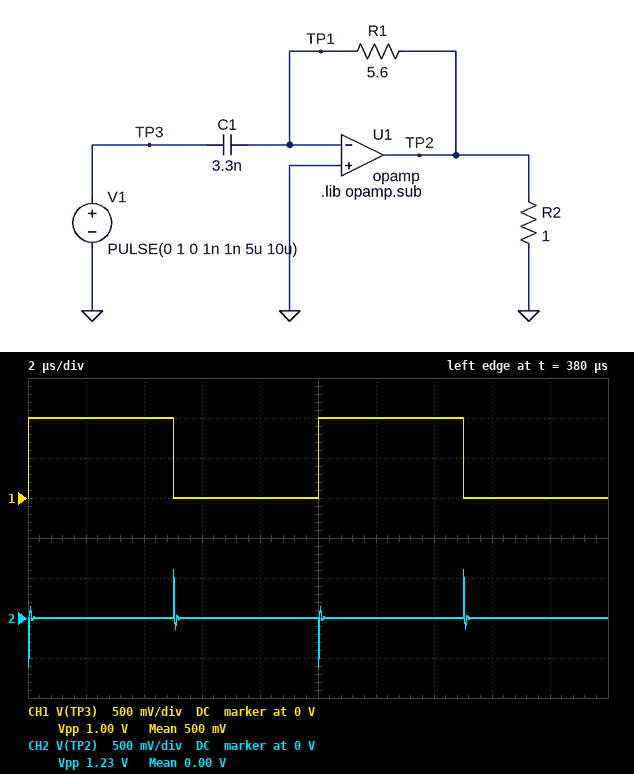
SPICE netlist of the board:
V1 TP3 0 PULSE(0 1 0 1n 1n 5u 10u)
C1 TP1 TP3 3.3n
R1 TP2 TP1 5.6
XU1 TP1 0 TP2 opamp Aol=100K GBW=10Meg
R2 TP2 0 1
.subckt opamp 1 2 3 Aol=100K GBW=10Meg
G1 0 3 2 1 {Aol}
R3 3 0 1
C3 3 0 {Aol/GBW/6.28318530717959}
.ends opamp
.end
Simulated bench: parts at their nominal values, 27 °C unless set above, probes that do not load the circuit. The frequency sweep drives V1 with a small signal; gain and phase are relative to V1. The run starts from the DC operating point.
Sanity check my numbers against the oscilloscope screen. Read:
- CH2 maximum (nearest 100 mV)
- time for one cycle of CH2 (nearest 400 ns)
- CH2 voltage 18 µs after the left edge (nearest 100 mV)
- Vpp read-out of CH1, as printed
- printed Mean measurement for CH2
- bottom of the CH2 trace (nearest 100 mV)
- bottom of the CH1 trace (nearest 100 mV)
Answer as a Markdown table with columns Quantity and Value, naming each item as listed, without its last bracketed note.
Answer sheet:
| Quantity | Value |
|---|---|
| CH2 maximum | 600 mV |
| time for one cycle of CH2 | 10.0 µs |
| CH2 voltage 18 µs after the left edge | 0 V |
| Vpp read-out of CH1, as printed | 1.00 V |
| printed Mean measurement for CH2 | 0.00 V |
| bottom of the CH2 trace | -600 mV |
| bottom of the CH1 trace | 0 V |
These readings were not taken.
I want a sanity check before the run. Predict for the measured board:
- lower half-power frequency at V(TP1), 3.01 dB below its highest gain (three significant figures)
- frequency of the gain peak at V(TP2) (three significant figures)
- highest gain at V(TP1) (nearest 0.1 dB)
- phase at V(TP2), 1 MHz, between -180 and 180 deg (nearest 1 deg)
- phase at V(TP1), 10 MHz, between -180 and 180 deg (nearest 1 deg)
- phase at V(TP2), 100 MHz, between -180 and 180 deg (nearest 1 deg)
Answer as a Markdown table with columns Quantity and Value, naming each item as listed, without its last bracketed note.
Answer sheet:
| Quantity | Value |
|---|---|
| lower half-power frequency at V(TP1), 3.01 dB below its highest gain | 7.87 MHz |
| frequency of the gain peak at V(TP2) | 9.28 MHz |
| highest gain at V(TP1) | 1.7 dB |
| phase at V(TP2), 1 MHz, between -180 and 180 deg | -96 deg |
| phase at V(TP1), 10 MHz, between -180 and 180 deg | 81 deg |
| phase at V(TP2), 100 MHz, between -180 and 180 deg | 95 deg |
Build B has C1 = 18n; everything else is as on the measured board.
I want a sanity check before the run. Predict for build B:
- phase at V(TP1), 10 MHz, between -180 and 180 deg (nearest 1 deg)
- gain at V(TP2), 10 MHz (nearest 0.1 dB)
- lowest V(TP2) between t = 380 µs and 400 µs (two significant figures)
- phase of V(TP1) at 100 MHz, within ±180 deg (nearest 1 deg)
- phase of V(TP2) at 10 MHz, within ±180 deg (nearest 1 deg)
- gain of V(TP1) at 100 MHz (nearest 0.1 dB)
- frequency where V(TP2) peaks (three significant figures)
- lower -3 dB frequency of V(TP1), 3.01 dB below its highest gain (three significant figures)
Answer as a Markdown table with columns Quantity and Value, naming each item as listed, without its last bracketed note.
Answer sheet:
| Quantity | Value |
|---|---|
| phase at V(TP1), 10 MHz, between -180 and 180 deg | 11 deg |
| gain at V(TP2), 10 MHz | 1.3 dB |
| lowest V(TP2) between t = 380 µs and 400 µs | -1.9 V |
| phase of V(TP1) at 100 MHz, within ±180 deg | 1 deg |
| phase of V(TP2) at 10 MHz, within ±180 deg | 101 deg |
| gain of V(TP1) at 100 MHz | 0 dB |
| frequency where V(TP2) peaks | 3.97 MHz |
| lower -3 dB frequency of V(TP1), 3.01 dB below its highest gain | 3.47 MHz |
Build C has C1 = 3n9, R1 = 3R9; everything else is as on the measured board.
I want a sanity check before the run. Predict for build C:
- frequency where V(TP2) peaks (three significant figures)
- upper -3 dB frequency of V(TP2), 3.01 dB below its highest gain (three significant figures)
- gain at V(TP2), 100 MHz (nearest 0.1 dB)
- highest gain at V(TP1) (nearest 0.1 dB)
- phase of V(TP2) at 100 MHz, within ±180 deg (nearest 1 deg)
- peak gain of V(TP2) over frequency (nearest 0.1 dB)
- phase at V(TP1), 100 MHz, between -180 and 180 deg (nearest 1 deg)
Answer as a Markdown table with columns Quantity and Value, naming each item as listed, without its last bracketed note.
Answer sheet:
| Quantity | Value |
|---|---|
| frequency where V(TP2) peaks | 10.2 MHz |
| upper -3 dB frequency of V(TP2), 3.01 dB below its highest gain | 16.7 MHz |
| gain at V(TP2), 100 MHz | -20.0 dB |
| highest gain at V(TP1) | 1.1 dB |
| phase of V(TP2) at 100 MHz, within ±180 deg | 96 deg |
| peak gain of V(TP2) over frequency | -0.4 dB |
| phase at V(TP1), 100 MHz, between -180 and 180 deg | 6 deg |
